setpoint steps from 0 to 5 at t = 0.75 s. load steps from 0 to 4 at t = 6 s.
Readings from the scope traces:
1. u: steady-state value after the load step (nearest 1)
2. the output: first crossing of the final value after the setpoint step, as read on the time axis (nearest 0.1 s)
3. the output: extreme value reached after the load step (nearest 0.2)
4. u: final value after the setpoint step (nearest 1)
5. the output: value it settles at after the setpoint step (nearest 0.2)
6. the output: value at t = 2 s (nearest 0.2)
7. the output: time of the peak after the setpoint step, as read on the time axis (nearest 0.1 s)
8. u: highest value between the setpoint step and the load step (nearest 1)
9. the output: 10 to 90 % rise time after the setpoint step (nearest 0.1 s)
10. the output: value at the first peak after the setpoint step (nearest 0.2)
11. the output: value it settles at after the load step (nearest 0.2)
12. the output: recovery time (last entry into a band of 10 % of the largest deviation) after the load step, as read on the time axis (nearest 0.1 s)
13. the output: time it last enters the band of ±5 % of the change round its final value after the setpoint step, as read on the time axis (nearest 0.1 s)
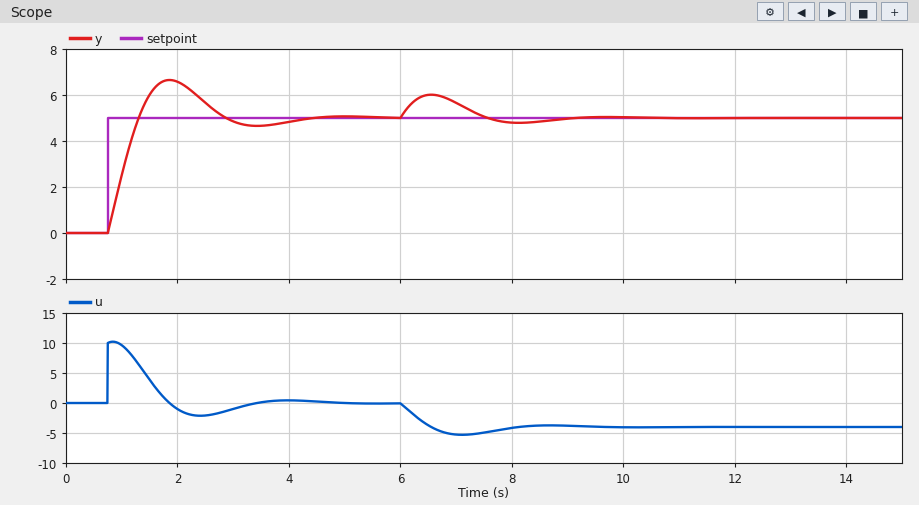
-4
1.3 s
6.0
0
5.0
6.6
1.9 s
10
0.4 s
6.6
5.0
8.7 s
3.8 s
